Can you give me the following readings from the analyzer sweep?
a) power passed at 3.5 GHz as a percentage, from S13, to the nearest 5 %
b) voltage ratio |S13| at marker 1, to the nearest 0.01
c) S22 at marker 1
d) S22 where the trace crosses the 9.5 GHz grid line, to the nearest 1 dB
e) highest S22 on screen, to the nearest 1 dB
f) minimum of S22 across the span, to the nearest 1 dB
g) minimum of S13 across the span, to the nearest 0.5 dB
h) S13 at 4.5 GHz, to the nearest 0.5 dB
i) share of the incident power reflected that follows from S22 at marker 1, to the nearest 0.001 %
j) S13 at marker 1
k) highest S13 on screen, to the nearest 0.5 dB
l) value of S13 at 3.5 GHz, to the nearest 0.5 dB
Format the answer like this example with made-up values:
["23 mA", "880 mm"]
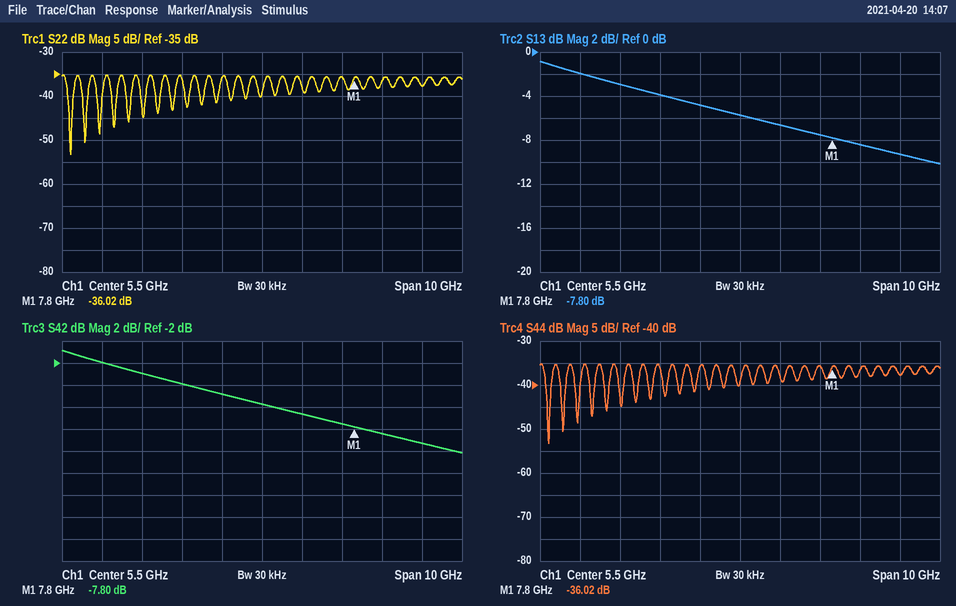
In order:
["40 %", "0.41", "-36.02 dB", "-38 dB", "-35 dB", "-53 dB", "-10.0 dB", "-5.0 dB", "0.025 %", "-7.80 dB", "-1.0 dB", "-4.0 dB"]
